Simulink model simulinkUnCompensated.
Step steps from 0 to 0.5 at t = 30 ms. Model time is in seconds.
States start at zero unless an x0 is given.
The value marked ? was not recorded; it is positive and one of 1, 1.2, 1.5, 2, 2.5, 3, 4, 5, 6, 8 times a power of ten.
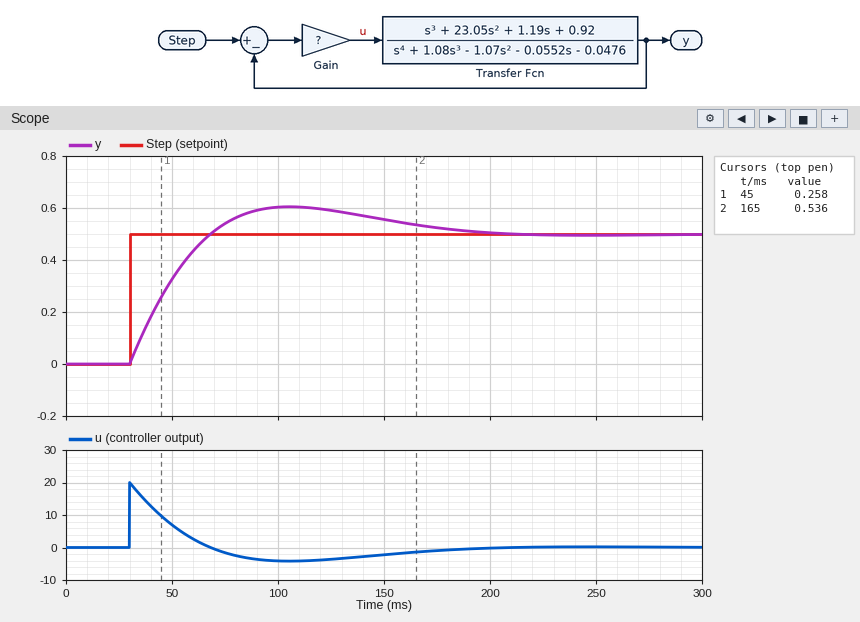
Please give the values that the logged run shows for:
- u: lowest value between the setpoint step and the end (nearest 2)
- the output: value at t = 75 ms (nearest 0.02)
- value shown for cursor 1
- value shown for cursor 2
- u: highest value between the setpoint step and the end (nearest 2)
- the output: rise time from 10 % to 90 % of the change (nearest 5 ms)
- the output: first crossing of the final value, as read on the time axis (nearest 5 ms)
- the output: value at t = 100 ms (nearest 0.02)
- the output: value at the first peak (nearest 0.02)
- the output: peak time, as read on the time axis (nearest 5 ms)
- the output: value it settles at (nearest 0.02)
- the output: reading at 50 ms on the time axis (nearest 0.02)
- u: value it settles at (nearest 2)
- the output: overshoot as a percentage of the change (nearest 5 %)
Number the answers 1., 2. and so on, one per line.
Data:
1. -4
2. 0.54
3. 0.258
4. 0.536
5. 20
6. 30 ms
7. 70 ms
8. 0.60
9. 0.60
10. 105 ms
11. 0.50
12. 0.32
13. 0
14. 20 %
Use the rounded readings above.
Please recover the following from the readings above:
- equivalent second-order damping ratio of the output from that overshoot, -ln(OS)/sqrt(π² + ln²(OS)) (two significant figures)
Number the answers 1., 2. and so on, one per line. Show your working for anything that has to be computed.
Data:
1. ln(0.2) = -1.609; 1.609 / sqrt(9.870 + 2.590) = 0.46
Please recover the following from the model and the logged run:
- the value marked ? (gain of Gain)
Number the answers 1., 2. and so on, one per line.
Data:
1. 40
